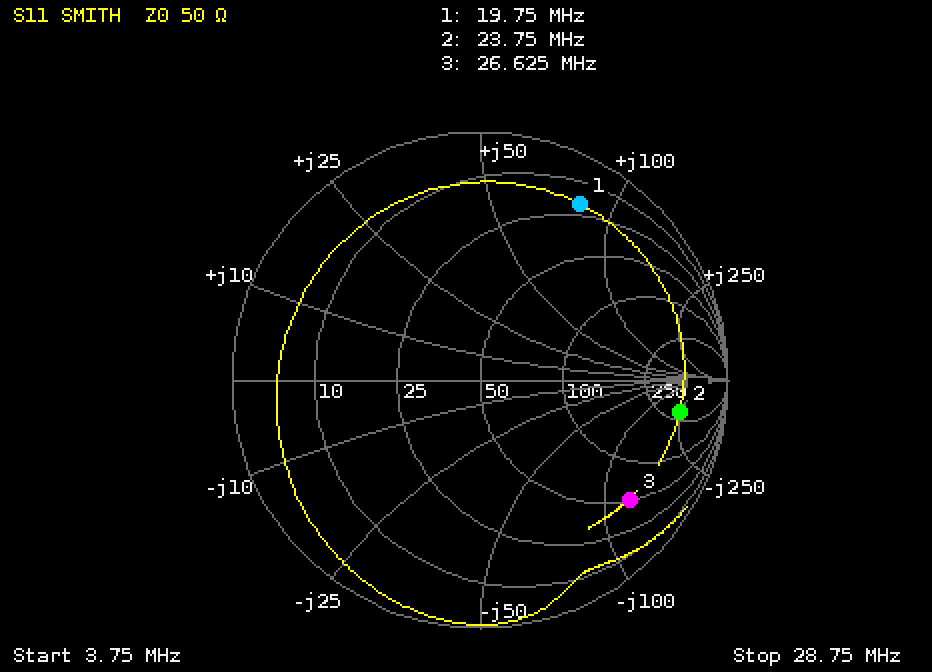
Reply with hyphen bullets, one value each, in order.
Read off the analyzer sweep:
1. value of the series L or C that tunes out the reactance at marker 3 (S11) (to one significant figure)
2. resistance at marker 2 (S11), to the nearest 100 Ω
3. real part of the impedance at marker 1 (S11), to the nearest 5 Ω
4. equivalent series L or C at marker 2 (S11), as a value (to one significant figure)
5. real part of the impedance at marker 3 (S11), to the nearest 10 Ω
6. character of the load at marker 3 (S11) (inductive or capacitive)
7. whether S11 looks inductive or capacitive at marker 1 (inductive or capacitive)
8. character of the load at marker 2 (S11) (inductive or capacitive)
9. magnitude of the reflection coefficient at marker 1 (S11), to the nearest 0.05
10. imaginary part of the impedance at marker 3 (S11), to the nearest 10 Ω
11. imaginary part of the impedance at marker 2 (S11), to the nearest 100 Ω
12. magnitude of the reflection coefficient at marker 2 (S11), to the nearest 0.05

- 700 nH
- 300 Ω
- 20 Ω
- 30 pF
- 50 Ω
- capacitive
- inductive
- capacitive
- 0.80
- -120 Ω
- -200 Ω
- 0.80
